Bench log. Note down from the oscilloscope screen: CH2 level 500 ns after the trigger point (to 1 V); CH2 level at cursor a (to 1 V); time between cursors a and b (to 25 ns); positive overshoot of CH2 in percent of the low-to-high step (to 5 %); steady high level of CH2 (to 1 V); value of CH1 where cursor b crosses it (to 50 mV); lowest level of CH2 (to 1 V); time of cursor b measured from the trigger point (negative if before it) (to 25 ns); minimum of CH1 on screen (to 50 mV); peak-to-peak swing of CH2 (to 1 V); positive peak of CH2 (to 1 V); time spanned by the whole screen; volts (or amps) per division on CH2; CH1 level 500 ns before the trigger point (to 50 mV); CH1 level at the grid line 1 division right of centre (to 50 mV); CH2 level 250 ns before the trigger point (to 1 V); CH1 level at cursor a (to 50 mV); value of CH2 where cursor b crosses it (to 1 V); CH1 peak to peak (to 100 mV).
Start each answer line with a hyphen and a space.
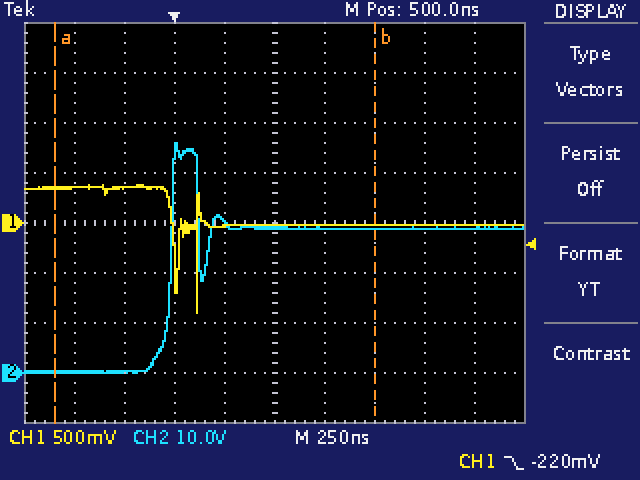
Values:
- 29 V
- 0 V
- 1.600 µs
- 60 %
- 29 V
- 0 mV
- 0 V
- +1.000 µs
- -900 mV
- 46 V
- 46 V
- 2.5 µs
- 10 V
- 350 mV
- 0 mV
- 0 V
- 350 mV
- 29 V
- 1.30 V
